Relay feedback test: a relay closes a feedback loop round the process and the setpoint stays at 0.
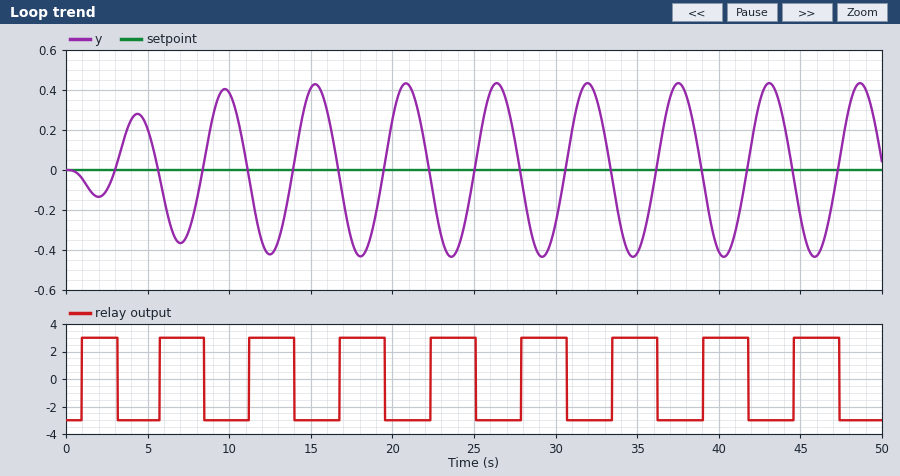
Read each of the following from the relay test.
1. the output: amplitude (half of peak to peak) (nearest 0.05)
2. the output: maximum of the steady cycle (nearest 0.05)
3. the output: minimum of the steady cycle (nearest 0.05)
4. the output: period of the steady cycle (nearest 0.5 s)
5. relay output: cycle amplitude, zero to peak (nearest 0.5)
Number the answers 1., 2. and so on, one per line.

1. 0.45
2. 0.45
3. -0.45
4. 5.5 s
5. 3.0
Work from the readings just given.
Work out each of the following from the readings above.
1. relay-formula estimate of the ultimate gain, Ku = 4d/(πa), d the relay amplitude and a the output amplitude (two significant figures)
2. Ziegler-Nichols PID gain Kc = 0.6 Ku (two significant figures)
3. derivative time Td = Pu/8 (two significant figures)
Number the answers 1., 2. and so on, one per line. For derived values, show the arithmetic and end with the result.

1. 4 × 3 / (π × 0.45) = 8.5
2. 0.6 × 8.5 = 5.1
3. 5.5 / 8 = 0.69 s
